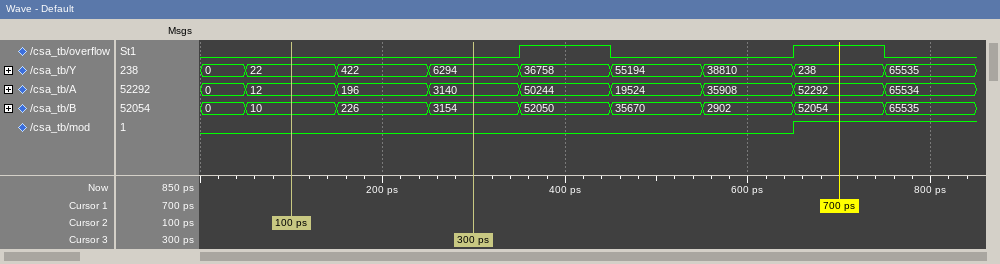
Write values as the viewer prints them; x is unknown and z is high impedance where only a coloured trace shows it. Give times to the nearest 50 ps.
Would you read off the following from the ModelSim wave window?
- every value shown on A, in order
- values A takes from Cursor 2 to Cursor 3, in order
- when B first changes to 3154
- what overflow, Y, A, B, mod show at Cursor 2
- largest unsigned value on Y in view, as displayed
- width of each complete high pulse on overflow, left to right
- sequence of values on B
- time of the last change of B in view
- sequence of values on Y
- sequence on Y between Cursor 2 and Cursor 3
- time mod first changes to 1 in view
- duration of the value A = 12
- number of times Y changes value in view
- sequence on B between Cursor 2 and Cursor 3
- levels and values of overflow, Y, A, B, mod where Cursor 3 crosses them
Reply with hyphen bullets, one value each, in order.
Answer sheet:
- 0, 12, 196, 3140, 50244, 19524, 35908, 52292, 65534
- 12, 196, 3140
- 250 ps
- overflow=0, Y=22, A=12, B=10, mod=0
- 65535
- 100 ps, 100 ps
- 0, 10, 226, 3154, 52050, 35670, 2902, 52054, 65535
- 750 ps
- 0, 22, 422, 6294, 36758, 55194, 38810, 238, 65535
- 22, 422, 6294
- 650 ps
- 100 ps
- 8
- 10, 226, 3154
- overflow=0, Y=6294, A=3140, B=3154, mod=0
